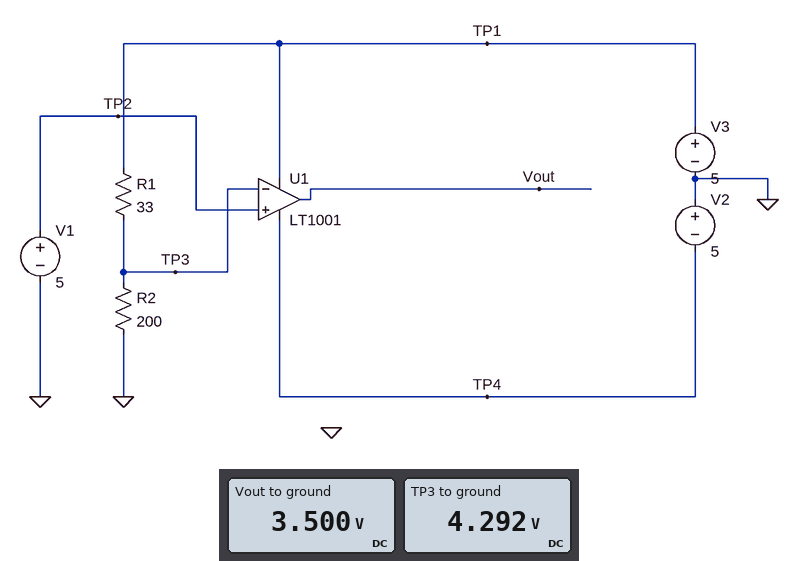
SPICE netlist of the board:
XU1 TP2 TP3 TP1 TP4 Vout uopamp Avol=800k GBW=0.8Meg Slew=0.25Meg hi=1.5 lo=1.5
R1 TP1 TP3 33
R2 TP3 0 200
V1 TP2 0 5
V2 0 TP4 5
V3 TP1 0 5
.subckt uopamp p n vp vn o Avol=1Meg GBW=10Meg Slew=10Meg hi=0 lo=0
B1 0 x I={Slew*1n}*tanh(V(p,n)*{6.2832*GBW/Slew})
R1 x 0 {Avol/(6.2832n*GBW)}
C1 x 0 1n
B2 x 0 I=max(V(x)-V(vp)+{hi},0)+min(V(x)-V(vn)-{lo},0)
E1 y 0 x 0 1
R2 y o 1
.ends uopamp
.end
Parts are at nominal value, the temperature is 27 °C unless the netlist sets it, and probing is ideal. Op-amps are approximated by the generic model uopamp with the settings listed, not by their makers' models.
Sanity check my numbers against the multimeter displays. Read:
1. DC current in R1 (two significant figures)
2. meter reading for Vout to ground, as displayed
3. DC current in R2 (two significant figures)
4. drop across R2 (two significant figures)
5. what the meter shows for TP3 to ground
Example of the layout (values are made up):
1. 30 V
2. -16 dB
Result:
1. 21 mA
2. 3.500 V
3. 21 mA
4. 4.3 V
5. 4.292 V
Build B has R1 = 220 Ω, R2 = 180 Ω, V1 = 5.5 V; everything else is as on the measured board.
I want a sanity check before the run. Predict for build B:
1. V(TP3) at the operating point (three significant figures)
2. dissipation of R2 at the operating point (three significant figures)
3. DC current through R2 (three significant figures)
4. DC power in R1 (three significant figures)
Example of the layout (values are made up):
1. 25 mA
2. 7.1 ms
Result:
1. 2.25 V
2. 28.1 mW
3. 12.5 mA
4. 34.4 mW
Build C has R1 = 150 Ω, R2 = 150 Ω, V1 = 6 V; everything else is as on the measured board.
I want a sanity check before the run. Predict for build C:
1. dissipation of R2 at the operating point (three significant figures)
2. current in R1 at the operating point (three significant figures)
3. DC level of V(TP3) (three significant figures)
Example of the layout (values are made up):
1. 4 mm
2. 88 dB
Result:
1. 41.7 mW
2. 16.7 mA
3. 2.50 V
